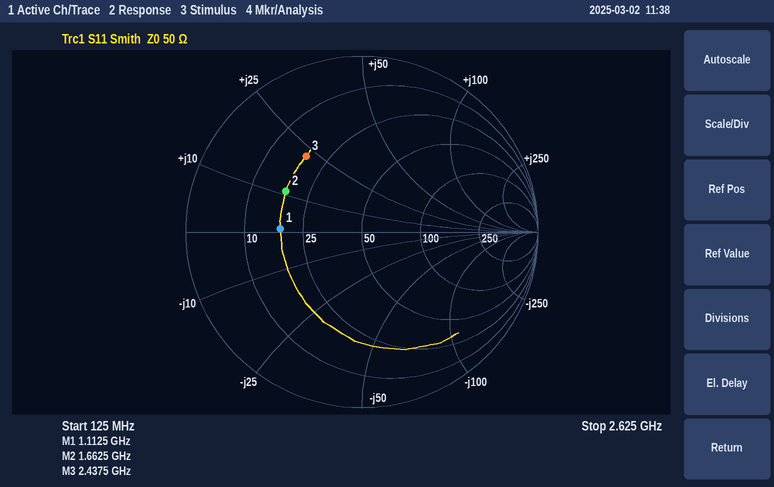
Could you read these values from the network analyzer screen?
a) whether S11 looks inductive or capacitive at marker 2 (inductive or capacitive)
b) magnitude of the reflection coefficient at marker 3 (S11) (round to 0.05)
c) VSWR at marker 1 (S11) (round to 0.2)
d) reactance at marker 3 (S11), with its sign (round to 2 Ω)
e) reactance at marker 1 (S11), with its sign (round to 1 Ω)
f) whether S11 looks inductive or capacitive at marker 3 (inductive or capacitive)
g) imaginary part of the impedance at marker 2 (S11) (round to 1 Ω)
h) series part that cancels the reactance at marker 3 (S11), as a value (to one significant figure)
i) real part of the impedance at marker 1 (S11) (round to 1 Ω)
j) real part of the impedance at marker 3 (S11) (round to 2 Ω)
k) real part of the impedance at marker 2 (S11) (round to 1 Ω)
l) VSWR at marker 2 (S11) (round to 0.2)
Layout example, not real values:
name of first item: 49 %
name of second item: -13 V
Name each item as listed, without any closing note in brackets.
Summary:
whether S11 looks inductive or capacitive at marker 2: inductive
magnitude of the reflection coefficient at marker 3 (S11): 0.55
VSWR at marker 1 (S11): 2.8
reactance at marker 3 (S11), with its sign: +22 Ω
reactance at marker 1 (S11), with its sign: +1 Ω
whether S11 looks inductive or capacitive at marker 3: inductive
imaginary part of the impedance at marker 2 (S11): +11 Ω
series part that cancels the reactance at marker 3 (S11), as a value: 3 pF
real part of the impedance at marker 1 (S11): 18 Ω
real part of the impedance at marker 3 (S11): 18 Ω
real part of the impedance at marker 2 (S11): 18 Ω
VSWR at marker 2 (S11): 3.0
